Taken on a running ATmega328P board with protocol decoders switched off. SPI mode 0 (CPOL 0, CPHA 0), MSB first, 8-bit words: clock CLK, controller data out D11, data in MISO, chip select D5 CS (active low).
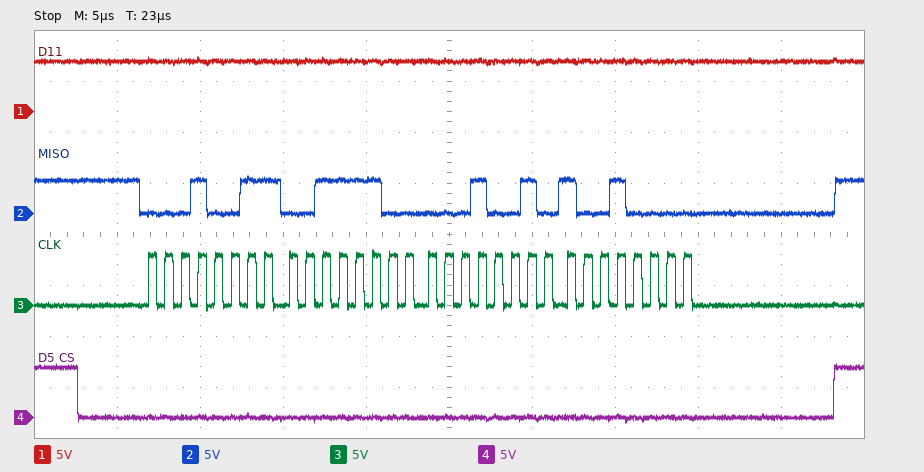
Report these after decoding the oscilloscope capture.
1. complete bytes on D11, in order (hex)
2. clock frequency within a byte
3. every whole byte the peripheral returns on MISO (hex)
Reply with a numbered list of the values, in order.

1. FF FF FF FF
2. 1 MHz
3. 13 3C 12 90
